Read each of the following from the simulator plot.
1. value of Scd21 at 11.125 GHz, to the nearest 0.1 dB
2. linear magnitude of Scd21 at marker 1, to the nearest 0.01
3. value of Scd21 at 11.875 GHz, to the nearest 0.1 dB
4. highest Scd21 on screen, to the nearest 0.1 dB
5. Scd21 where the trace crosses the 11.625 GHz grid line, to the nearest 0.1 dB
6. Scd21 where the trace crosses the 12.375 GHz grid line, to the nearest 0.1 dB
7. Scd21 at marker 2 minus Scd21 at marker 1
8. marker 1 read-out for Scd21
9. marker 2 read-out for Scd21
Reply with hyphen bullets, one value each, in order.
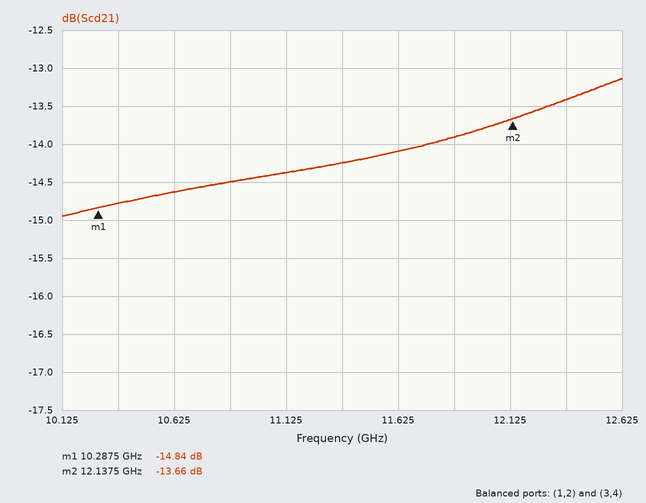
- -14.4 dB
- 0.18
- -13.9 dB
- -13.1 dB
- -14.1 dB
- -13.4 dB
- 1.18 dB
- -14.84 dB
- -13.66 dB
